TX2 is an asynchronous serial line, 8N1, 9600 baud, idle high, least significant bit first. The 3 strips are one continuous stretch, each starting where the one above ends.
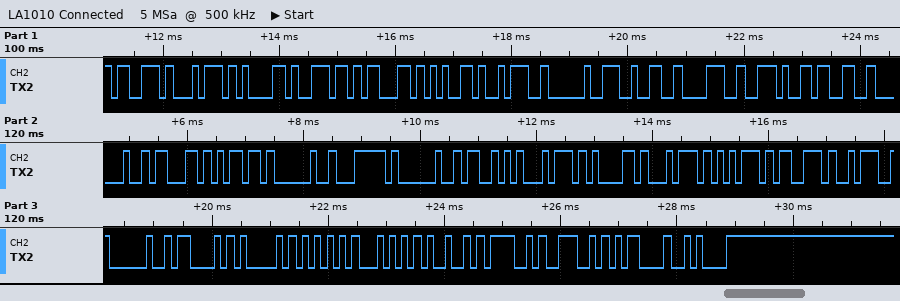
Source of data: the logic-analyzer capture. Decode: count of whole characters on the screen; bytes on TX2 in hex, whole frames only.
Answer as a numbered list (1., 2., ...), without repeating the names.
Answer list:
1. 35
2. 0x73 0x74 0x61 0x6E 0x63 0x65 0x3A 0x20 0x32 0x38 0x2E 0x33 0x20 0x63 0x6D 0x20 0x7C 0x20 0x53 0x74 0x61 0x74 0x75 0x73 0x3A 0x20 0x43 0x41 0x55 0x54 0x49 0x4F 0x4E 0x0D 0x0A
